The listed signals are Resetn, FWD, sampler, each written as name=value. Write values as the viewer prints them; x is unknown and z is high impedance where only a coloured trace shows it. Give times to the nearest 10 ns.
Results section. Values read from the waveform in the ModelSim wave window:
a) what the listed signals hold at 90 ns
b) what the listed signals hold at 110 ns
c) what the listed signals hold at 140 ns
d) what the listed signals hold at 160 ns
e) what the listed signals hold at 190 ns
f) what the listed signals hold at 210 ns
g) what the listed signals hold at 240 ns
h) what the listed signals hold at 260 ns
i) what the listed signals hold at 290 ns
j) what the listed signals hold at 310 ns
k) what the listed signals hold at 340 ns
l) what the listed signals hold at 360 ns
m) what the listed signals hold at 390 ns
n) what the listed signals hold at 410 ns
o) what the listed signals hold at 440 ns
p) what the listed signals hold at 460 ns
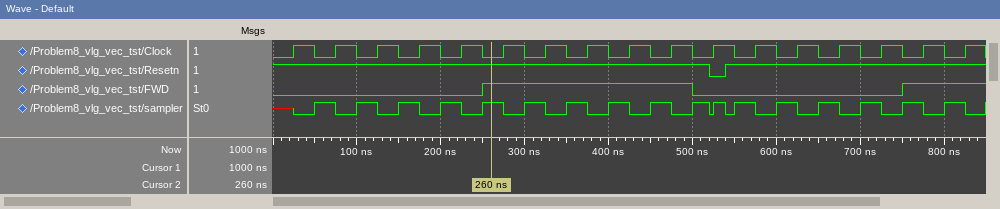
Resetn=1, FWD=0, sampler=0
Resetn=1, FWD=0, sampler=1
Resetn=1, FWD=0, sampler=0
Resetn=1, FWD=0, sampler=1
Resetn=1, FWD=0, sampler=0
Resetn=1, FWD=0, sampler=1
Resetn=1, FWD=0, sampler=0
Resetn=1, FWD=1, sampler=1
Resetn=1, FWD=1, sampler=0
Resetn=1, FWD=1, sampler=1
Resetn=1, FWD=1, sampler=0
Resetn=1, FWD=1, sampler=1
Resetn=1, FWD=1, sampler=0
Resetn=1, FWD=1, sampler=1
Resetn=1, FWD=1, sampler=0
Resetn=1, FWD=1, sampler=1
